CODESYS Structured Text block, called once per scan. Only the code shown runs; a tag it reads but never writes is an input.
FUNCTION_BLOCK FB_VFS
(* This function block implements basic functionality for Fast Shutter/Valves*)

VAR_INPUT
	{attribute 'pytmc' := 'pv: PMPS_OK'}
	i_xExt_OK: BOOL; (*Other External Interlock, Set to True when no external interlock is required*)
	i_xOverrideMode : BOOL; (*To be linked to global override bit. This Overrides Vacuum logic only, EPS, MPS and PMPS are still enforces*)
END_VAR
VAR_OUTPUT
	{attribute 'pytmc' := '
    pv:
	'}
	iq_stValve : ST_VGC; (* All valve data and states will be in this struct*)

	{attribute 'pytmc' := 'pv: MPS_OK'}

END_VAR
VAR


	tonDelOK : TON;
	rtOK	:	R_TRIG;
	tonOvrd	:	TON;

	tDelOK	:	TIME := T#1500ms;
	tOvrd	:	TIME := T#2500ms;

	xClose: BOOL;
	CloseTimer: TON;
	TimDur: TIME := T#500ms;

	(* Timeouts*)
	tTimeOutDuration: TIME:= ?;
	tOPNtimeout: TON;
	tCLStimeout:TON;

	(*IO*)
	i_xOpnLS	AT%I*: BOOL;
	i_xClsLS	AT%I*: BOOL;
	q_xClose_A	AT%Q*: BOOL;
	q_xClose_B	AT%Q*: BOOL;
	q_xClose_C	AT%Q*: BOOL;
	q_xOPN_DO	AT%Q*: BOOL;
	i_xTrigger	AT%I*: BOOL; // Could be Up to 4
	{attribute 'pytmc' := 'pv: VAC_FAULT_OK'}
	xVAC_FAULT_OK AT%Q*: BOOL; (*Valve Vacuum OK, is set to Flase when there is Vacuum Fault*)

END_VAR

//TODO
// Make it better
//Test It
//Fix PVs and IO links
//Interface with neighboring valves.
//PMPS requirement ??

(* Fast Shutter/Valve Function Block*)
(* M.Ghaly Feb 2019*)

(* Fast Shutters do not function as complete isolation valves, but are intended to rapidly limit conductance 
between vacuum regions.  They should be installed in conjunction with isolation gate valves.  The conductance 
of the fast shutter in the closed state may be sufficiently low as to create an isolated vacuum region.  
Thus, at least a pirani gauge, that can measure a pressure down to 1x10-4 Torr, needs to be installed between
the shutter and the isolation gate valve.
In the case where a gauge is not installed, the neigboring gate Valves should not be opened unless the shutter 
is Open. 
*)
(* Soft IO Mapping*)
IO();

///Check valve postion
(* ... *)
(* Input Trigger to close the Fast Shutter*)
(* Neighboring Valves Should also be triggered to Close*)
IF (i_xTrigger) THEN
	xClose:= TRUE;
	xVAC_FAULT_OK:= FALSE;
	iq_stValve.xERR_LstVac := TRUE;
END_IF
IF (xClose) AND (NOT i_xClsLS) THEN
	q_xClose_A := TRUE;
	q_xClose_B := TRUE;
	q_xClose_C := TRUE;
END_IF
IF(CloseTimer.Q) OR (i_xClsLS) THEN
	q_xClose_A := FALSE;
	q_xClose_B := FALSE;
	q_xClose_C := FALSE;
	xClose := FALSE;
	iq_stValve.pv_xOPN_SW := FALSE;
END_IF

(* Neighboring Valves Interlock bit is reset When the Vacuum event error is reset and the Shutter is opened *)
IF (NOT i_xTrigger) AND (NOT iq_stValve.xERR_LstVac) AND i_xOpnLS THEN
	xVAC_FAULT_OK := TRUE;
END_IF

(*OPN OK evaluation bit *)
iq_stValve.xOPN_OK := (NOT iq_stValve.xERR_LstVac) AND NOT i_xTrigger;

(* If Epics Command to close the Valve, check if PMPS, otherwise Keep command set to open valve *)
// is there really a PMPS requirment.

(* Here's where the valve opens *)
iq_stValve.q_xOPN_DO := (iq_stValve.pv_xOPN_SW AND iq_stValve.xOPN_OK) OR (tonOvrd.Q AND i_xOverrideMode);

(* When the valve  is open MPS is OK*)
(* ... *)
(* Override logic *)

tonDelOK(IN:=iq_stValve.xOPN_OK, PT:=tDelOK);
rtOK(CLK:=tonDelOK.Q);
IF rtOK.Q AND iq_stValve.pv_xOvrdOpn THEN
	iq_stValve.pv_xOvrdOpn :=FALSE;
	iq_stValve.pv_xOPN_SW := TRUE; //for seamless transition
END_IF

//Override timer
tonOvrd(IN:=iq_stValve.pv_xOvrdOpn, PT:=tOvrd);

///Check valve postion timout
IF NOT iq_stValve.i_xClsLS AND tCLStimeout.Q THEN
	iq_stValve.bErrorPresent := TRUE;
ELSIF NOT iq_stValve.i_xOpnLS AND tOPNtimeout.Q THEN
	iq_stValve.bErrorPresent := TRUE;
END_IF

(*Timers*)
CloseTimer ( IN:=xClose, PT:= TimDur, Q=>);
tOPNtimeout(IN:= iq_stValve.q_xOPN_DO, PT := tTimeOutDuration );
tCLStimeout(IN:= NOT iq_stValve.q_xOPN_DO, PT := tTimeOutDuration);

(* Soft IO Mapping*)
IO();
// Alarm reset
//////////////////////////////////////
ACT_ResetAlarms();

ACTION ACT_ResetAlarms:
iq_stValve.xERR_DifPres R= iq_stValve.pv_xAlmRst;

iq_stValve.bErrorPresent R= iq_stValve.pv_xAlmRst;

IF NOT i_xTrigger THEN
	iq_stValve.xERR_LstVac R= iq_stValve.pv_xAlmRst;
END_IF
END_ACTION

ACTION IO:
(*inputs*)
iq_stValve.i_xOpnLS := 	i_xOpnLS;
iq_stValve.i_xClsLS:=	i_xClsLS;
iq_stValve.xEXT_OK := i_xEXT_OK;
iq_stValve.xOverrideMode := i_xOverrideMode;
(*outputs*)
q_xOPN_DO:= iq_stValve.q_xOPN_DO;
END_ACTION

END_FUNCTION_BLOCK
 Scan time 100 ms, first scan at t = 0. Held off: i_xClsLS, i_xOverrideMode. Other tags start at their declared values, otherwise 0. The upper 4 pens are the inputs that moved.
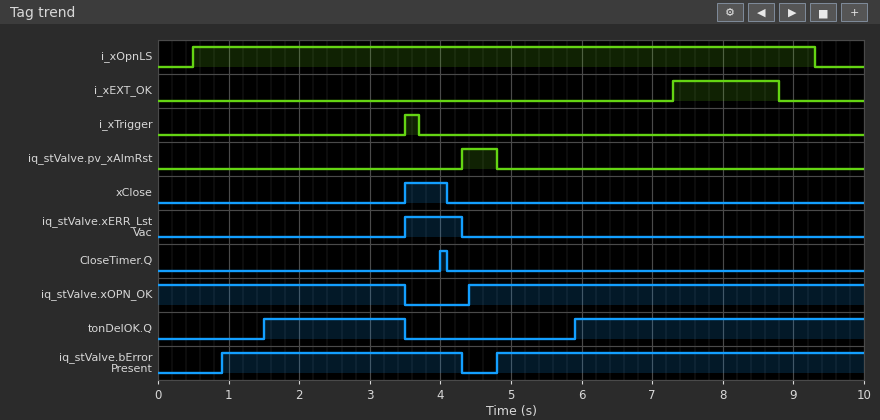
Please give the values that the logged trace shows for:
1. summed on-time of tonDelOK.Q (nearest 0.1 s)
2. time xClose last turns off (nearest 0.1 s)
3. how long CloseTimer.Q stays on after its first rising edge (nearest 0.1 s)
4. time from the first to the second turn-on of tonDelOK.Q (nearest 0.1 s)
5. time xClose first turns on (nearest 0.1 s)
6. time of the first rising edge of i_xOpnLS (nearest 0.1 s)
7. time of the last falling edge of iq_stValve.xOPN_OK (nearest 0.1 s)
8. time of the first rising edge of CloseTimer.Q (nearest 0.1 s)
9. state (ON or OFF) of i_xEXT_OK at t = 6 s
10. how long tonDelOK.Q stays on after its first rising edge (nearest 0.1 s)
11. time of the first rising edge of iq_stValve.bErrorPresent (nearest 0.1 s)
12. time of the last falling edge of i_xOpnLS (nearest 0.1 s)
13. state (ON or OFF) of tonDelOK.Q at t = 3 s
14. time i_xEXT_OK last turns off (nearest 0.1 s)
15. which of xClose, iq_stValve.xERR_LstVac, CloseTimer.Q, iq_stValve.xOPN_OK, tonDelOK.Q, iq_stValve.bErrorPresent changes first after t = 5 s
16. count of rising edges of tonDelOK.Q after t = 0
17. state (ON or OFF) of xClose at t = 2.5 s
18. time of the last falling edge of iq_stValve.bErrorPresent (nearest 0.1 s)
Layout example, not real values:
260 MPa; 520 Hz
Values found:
6.1 s; 4.1 s; 0.1 s; 4.4 s; 3.5 s; 0.5 s; 3.5 s; 4.0 s; OFF; 2.0 s; 0.9 s; 9.3 s; ON; 8.8 s; tonDelOK.Q; 2; OFF; 4.3 s
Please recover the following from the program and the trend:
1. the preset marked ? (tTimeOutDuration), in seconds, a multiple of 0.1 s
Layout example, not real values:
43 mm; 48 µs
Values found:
0.8 s
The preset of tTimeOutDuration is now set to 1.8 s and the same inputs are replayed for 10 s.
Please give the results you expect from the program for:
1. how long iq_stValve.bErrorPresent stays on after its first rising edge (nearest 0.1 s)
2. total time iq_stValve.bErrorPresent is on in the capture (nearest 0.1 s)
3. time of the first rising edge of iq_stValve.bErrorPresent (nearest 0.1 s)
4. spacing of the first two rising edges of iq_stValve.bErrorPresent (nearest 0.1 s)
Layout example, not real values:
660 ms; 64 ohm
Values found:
2.4 s; 7.6 s; 1.9 s; 2.9 s
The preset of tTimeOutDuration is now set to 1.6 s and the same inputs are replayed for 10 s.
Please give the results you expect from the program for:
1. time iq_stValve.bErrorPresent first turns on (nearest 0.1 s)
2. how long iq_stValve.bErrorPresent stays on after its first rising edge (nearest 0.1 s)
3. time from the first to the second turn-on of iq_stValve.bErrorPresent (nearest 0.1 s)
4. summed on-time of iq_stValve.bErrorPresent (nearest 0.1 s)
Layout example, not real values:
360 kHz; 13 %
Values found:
1.7 s; 2.6 s; 3.1 s; 7.8 s
